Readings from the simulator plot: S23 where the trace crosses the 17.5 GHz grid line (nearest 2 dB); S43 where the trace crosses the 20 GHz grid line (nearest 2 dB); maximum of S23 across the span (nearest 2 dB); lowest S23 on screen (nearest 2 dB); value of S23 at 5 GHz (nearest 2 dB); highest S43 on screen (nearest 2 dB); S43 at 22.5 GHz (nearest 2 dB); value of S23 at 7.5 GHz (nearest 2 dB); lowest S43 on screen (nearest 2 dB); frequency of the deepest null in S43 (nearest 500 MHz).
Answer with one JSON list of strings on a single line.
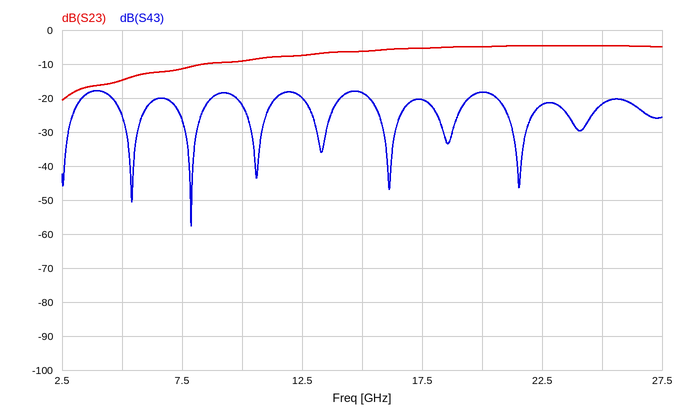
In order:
["-6 dB", "-18 dB", "-4 dB", "-20 dB", "-14 dB", "-18 dB", "-22 dB", "-12 dB", "-58 dB", "8.0 GHz"]
